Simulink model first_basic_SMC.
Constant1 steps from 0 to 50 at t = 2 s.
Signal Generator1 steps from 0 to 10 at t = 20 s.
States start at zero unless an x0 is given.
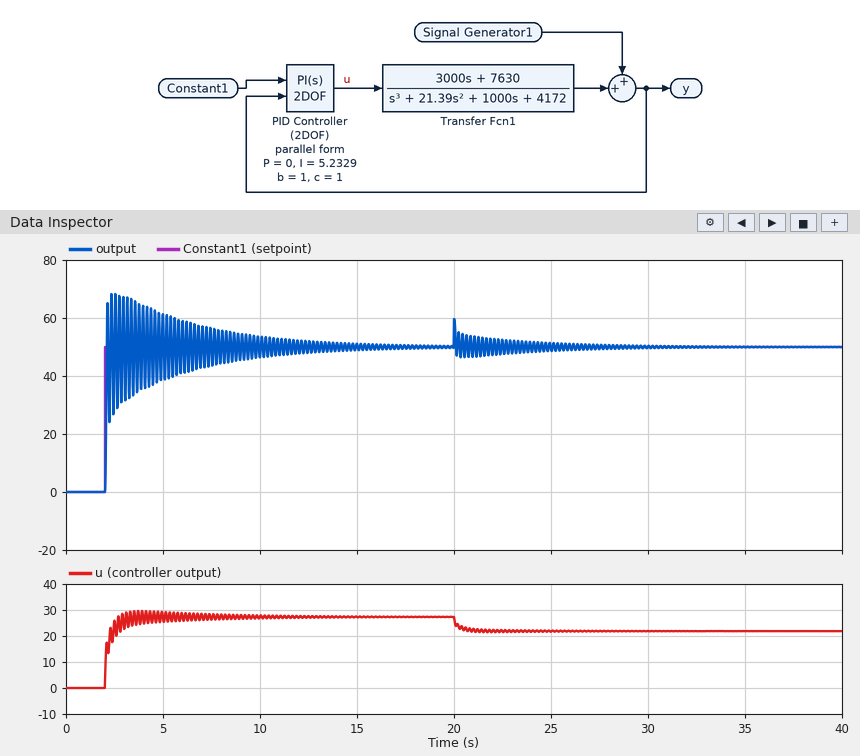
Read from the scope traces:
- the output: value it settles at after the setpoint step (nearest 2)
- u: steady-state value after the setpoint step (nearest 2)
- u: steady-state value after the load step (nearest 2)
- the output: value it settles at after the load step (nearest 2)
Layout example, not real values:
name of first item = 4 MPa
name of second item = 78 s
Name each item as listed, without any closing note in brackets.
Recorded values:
the output: value it settles at after the setpoint step = 50
u: steady-state value after the setpoint step = 28
u: steady-state value after the load step = 22
the output: value it settles at after the load step = 50
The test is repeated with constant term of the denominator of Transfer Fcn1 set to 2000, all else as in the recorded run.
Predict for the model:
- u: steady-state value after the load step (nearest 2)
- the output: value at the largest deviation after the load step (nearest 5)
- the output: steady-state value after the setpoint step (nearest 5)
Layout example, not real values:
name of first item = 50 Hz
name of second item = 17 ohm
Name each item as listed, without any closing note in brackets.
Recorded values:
u: steady-state value after the load step = 10
the output: value at the largest deviation after the load step = 60
the output: steady-state value after the setpoint step = 50
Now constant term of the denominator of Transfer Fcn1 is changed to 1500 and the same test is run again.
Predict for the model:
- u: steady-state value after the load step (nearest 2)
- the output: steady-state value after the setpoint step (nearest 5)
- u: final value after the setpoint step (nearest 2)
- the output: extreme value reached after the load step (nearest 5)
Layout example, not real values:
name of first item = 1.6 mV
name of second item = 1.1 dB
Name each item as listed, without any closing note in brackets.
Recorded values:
u: steady-state value after the load step = 8
the output: steady-state value after the setpoint step = 50
u: final value after the setpoint step = 10
the output: extreme value reached after the load step = 60
